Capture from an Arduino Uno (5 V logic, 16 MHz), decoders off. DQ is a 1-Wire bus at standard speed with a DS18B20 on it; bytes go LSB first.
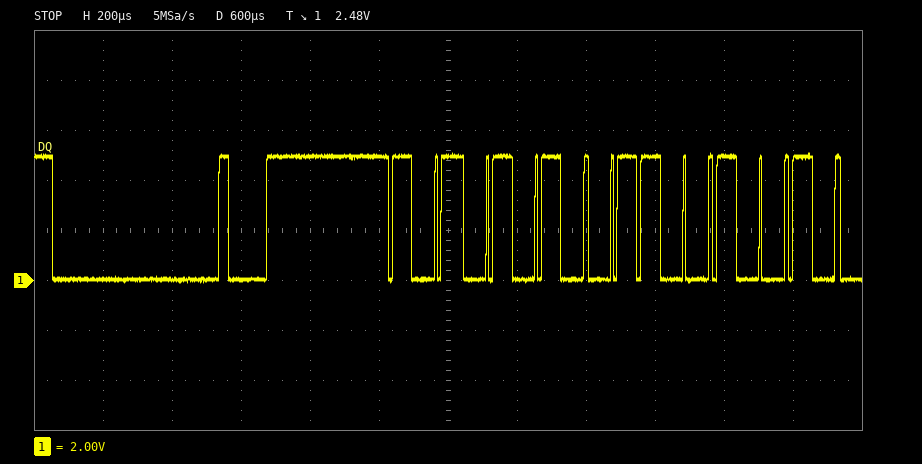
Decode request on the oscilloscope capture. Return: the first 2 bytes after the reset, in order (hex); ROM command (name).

55 26
Match ROM
